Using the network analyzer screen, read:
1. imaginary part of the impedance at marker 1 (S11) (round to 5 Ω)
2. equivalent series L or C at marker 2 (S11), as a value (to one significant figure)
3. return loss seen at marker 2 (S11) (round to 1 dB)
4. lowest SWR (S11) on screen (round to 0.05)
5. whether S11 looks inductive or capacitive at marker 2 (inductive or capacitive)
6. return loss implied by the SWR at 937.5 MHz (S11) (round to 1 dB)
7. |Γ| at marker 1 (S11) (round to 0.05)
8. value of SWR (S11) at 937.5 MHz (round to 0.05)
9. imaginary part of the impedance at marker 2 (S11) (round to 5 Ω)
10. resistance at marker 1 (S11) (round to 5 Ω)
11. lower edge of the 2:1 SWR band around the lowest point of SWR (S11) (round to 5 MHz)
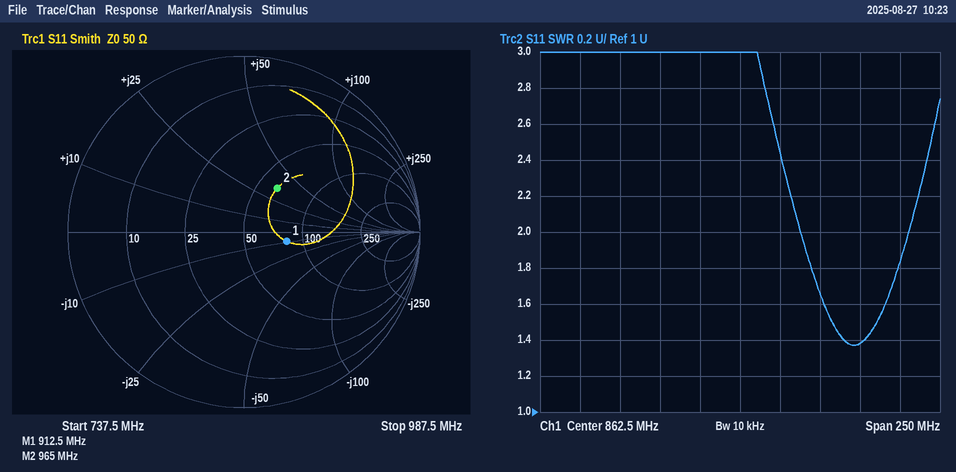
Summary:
-10 Ω
6 nH
10 dB
1.35
inductive
16 dB
0.25
1.40
+35 Ω
80 Ω
900 MHz
